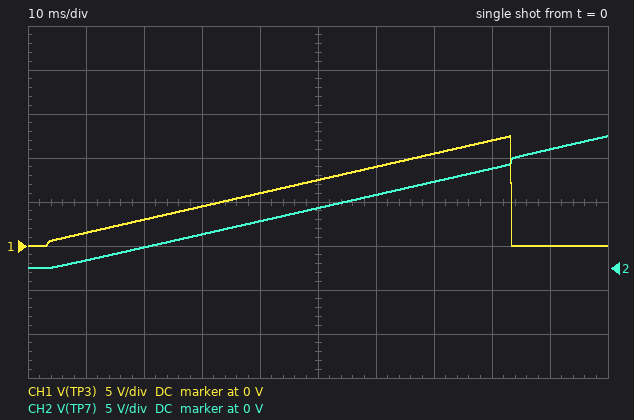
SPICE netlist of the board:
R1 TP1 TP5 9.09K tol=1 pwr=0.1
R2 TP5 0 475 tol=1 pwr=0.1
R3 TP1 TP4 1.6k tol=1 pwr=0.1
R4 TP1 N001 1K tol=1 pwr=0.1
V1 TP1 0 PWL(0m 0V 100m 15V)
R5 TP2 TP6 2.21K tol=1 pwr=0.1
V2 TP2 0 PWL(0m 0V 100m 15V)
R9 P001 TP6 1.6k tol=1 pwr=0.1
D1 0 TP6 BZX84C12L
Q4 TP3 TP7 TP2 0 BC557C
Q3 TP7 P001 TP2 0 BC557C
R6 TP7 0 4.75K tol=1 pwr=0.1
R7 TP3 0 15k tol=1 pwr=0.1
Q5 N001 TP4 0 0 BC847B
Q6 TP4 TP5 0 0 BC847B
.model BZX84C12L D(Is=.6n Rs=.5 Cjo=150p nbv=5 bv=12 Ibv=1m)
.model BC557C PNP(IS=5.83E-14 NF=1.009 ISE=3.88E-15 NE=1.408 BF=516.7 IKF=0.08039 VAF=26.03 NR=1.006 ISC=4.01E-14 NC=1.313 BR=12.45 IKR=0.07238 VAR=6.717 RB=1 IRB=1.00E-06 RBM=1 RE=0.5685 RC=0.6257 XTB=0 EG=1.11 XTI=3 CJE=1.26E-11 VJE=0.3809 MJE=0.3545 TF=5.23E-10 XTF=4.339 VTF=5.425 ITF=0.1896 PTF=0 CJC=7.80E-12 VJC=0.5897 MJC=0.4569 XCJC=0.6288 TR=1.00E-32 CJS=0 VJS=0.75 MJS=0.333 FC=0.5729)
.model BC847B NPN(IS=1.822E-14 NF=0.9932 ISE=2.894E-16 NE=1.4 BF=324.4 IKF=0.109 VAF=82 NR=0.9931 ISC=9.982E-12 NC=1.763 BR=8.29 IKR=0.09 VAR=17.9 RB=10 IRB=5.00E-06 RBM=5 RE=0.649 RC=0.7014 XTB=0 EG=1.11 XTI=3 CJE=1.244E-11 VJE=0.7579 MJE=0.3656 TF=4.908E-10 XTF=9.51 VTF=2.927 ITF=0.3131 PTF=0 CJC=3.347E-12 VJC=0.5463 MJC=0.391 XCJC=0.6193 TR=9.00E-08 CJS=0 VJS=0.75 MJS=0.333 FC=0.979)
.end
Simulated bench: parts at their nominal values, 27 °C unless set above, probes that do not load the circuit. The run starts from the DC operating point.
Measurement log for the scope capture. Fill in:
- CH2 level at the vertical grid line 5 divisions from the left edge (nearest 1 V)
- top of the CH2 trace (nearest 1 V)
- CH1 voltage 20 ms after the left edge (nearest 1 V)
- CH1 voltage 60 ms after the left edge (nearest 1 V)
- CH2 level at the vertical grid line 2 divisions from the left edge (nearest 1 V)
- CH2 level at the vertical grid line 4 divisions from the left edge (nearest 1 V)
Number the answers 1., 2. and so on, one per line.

1. 7 V
2. 15 V
3. 3 V
4. 9 V
5. 2 V
6. 5 V
